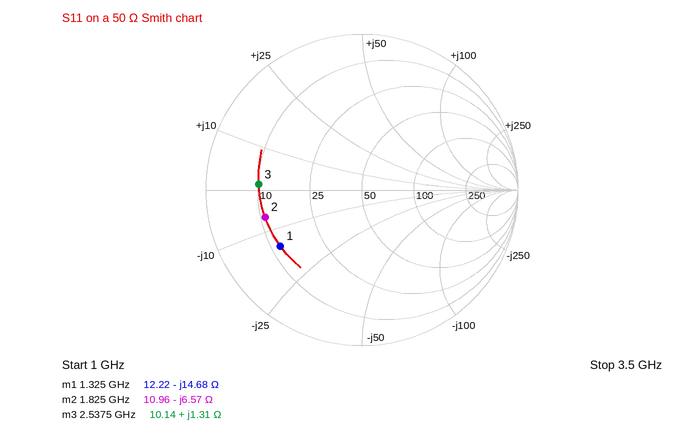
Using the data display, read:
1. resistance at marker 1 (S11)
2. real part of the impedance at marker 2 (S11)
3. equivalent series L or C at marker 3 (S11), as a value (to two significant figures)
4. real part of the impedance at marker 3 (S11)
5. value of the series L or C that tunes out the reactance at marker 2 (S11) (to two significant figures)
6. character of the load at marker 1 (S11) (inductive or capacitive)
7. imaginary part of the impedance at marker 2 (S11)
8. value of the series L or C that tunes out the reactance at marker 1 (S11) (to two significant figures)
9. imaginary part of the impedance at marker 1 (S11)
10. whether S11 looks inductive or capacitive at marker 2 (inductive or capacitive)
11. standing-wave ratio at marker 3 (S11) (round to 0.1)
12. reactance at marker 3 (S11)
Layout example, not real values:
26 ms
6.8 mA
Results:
12.22 Ω
10.96 Ω
82 pH
10.14 Ω
570 pH
capacitive
-6.57 Ω
1.8 nH
-14.68 Ω
capacitive
4.9
+1.31 Ω
